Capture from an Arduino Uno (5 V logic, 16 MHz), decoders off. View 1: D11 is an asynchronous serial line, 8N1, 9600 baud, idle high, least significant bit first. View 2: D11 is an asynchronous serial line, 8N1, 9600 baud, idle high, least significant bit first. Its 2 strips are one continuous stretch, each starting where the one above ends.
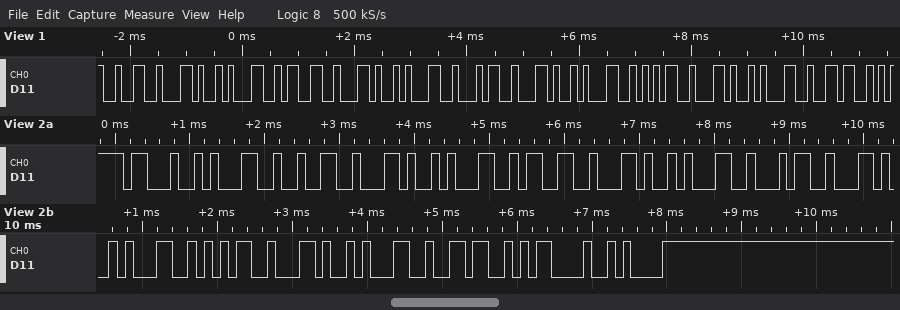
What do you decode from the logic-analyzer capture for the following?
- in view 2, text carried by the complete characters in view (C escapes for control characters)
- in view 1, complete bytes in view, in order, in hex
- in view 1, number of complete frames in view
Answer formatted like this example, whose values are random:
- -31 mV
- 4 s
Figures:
- "#12,13,14,15,16\r\n"
- 32 2C 31 33 2C 31 34 2C 31 35 2C 31 36
- 13
